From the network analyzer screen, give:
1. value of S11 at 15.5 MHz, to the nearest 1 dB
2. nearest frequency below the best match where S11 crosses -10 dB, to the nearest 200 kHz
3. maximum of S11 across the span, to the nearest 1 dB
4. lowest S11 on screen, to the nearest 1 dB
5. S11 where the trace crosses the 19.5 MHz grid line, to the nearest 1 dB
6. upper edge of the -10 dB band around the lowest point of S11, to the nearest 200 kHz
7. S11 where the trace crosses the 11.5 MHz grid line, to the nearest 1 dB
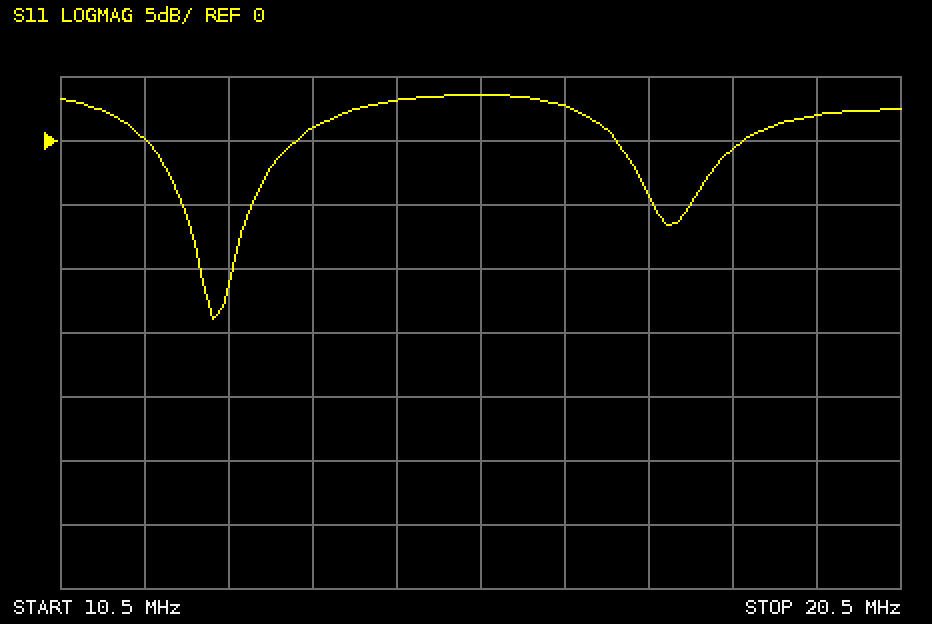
4 dB
12.2 MHz
4 dB
-14 dB
2 dB
12.6 MHz
0 dB
